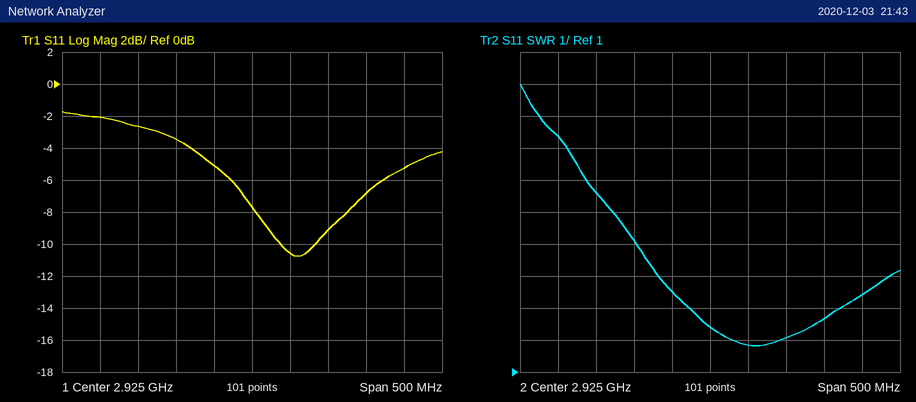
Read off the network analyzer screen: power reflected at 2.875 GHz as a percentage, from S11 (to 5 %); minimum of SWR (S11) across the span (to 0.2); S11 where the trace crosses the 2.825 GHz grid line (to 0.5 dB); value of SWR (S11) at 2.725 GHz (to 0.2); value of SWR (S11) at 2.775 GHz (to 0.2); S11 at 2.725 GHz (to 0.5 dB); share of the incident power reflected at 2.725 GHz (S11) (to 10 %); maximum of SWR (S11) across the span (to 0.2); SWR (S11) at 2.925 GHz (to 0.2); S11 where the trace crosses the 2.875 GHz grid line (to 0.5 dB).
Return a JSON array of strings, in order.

["30 %", "1.8", "-3.5 dB", "8.4", "6.6", "-2.0 dB", "60 %", "10.0", "2.4", "-5.0 dB"]
